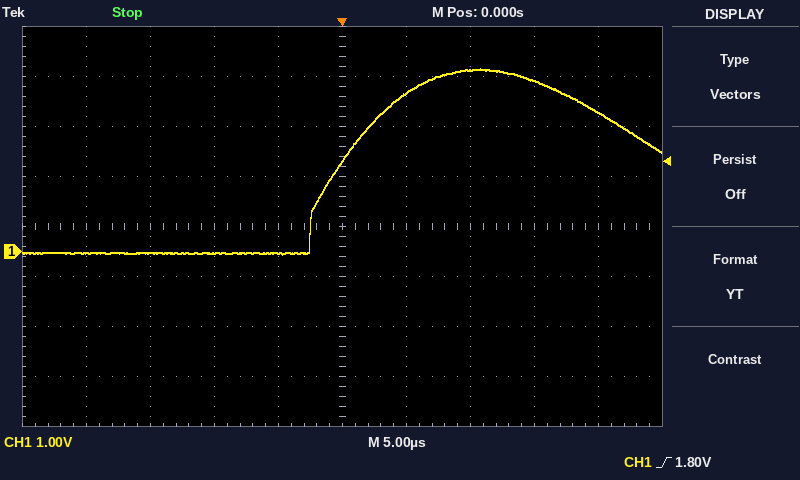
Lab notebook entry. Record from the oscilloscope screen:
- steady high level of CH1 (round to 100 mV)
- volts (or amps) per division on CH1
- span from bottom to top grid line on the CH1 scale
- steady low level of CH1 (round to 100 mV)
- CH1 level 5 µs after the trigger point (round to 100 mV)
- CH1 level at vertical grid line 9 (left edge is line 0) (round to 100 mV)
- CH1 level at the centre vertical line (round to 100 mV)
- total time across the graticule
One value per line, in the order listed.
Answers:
3.6 V
1 V
8 V
0.0 V
3.2 V
2.8 V
1.8 V
50 µs
